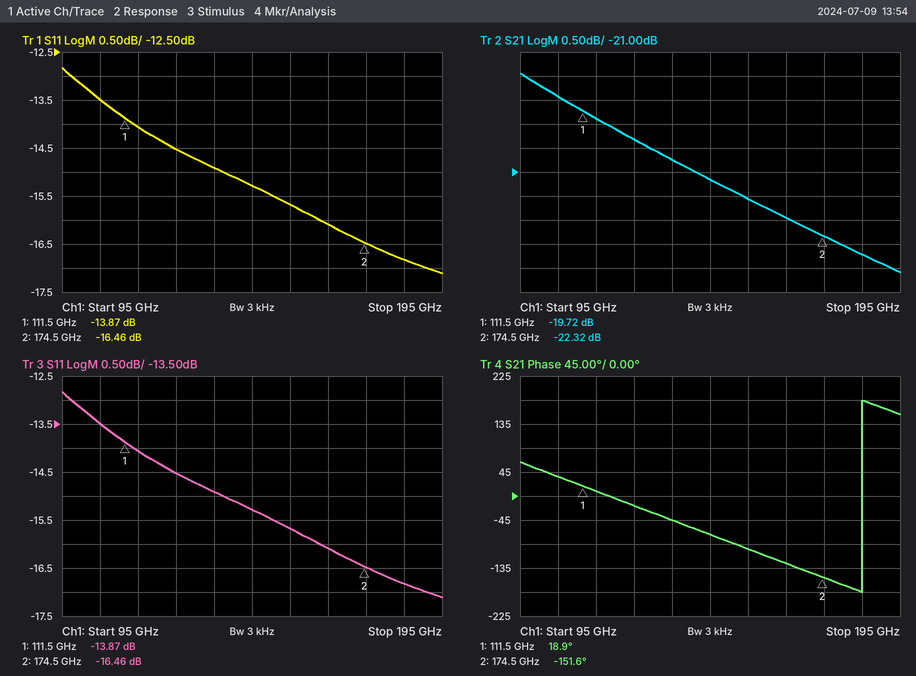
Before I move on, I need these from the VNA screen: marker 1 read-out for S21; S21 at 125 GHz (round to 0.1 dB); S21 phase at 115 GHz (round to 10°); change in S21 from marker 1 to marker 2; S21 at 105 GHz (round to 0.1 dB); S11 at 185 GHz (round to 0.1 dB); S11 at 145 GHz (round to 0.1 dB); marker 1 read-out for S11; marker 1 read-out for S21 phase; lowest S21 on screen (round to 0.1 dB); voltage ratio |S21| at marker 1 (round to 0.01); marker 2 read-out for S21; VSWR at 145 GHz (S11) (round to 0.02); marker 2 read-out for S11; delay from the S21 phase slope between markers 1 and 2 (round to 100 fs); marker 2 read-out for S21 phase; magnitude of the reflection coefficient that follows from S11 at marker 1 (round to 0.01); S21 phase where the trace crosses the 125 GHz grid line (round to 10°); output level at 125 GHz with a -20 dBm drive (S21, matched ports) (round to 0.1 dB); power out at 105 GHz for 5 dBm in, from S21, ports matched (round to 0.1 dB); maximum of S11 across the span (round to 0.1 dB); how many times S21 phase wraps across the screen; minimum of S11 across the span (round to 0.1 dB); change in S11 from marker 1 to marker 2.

-19.72 dB
-20.3 dB
10°
-2.60 dB
-19.4 dB
-16.8 dB
-15.3 dB
-13.87 dB
18.9°
-23.1 dB
0.10
-22.32 dB
1.42
-16.46 dB
7.5 ps
-151.6°
0.20
-20°
-40.3 dBm
-14.4 dBm
-12.8 dB
1
-17.1 dB
-2.59 dB
